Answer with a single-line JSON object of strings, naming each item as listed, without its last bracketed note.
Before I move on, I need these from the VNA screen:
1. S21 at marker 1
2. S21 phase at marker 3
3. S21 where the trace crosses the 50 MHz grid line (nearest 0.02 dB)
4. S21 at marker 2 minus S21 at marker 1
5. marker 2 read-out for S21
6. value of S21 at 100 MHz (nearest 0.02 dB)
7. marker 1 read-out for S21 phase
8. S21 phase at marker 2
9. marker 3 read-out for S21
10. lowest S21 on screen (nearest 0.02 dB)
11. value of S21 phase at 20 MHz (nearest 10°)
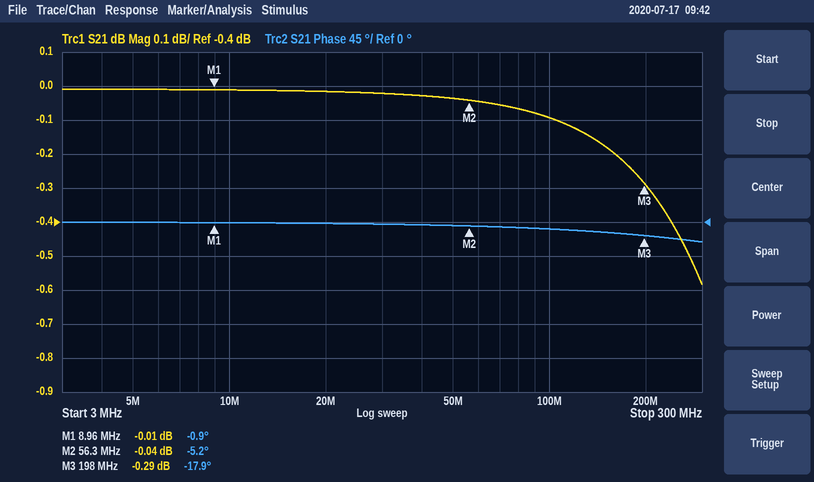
{"S21 at marker 1": "-0.01 dB", "S21 phase at marker 3": "-17.9°", "S21 where the trace crosses the 50 MHz grid line": "-0.04 dB", "S21 at marker 2 minus S21 at marker 1": "-0.03 dB", "marker 2 read-out for S21": "-0.04 dB", "value of S21 at 100 MHz": "-0.10 dB", "marker 1 read-out for S21 phase": "-0.9°", "S21 phase at marker 2": "-5.2°", "marker 3 read-out for S21": "-0.29 dB", "lowest S21 on screen": "-0.58 dB", "value of S21 phase at 20 MHz": "0°"}
